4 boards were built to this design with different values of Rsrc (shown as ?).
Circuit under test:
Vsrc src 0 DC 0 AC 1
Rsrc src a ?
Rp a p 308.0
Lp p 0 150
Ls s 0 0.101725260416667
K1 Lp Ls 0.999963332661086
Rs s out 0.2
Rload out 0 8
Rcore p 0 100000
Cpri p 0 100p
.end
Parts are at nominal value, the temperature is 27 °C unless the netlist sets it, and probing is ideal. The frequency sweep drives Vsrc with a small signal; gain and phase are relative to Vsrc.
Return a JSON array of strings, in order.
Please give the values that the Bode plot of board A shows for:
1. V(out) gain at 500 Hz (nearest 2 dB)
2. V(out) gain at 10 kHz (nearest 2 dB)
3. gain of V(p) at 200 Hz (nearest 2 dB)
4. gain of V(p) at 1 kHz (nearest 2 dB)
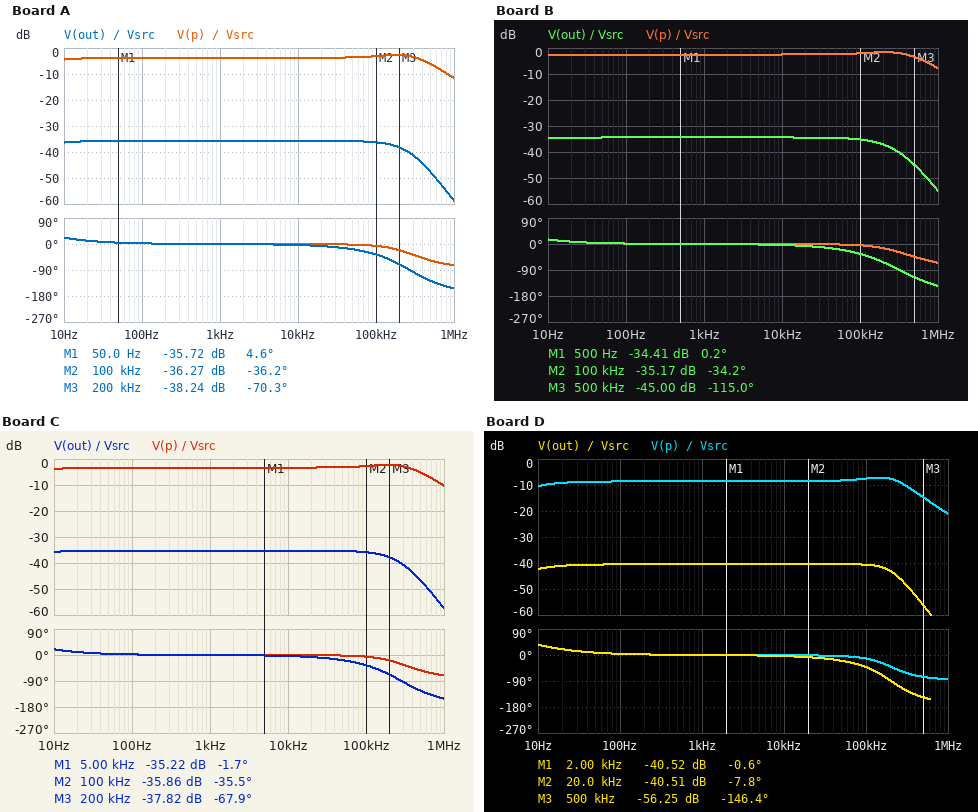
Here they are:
["-36 dB", "-36 dB", "-4 dB", "-4 dB"]
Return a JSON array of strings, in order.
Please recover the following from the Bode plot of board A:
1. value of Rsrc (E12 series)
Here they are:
["5.6 kΩ"]
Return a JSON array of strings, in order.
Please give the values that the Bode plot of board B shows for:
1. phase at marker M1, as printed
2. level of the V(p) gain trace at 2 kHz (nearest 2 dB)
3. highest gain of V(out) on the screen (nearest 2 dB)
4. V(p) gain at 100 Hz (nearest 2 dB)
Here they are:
["0.2 deg", "-2 dB", "-34 dB", "-2 dB"]
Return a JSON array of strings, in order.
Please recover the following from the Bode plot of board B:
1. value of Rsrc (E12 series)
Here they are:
["3.3 kΩ"]
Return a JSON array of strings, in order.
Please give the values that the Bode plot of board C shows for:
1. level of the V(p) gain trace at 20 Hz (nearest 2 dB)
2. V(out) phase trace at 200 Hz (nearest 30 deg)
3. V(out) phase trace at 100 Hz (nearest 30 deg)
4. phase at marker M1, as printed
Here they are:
["-4 dB", "0 deg", "0 deg", "-1.7 deg"]
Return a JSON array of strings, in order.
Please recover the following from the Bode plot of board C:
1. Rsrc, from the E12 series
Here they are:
["4.7 kΩ"]
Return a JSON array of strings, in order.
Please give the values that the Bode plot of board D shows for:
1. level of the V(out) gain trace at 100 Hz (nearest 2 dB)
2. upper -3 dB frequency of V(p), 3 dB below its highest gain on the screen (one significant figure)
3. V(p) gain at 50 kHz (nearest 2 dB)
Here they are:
["-40 dB", "300 kHz", "-8 dB"]
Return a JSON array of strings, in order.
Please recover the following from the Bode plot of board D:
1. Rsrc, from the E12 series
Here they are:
["18 kΩ"]
